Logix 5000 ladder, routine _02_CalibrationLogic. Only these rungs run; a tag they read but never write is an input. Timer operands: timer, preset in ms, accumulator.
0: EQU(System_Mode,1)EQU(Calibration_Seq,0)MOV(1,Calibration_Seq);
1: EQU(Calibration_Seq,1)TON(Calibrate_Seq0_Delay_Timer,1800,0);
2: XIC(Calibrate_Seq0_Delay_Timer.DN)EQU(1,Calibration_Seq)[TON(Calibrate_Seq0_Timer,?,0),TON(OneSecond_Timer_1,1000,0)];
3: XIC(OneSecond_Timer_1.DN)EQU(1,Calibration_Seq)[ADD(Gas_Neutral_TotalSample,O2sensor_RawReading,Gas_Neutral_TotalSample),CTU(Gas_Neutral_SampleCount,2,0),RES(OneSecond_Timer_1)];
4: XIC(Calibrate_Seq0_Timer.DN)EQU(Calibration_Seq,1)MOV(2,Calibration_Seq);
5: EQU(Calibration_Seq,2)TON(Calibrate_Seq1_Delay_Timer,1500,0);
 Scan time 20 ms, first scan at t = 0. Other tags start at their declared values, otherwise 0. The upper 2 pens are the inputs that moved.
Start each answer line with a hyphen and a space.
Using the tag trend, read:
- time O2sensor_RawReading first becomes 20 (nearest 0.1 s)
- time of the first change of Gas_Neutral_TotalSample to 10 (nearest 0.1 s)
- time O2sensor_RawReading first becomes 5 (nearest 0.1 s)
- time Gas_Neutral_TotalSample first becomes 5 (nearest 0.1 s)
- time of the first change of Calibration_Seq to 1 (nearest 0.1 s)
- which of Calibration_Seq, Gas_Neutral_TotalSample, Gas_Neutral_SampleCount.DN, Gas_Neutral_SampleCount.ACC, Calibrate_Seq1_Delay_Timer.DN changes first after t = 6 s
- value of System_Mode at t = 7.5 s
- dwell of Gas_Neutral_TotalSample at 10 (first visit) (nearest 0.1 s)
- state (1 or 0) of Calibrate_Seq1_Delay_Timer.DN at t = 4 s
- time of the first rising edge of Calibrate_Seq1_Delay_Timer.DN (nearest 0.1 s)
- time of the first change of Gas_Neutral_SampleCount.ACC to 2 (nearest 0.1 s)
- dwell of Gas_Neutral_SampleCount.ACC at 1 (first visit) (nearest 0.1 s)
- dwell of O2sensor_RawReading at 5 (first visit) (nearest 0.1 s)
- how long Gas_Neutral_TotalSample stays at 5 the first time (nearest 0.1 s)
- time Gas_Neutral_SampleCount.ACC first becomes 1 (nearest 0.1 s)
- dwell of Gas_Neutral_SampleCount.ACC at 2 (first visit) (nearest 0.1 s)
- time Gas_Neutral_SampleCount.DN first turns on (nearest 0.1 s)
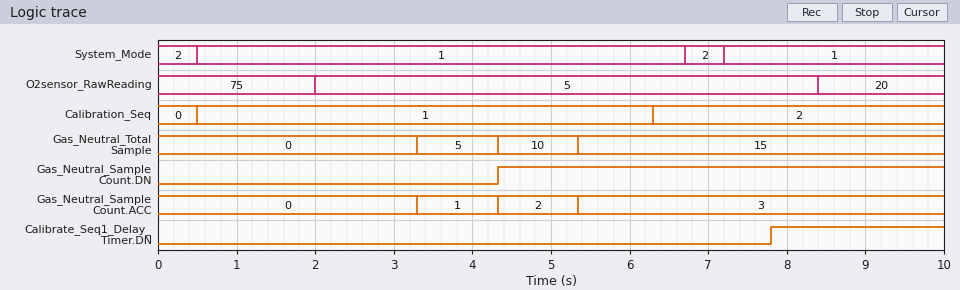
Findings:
- 8.4 s
- 4.3 s
- 2.0 s
- 3.3 s
- 0.5 s
- Calibration_Seq
- 1
- 1.0 s
- 0
- 7.8 s
- 4.3 s
- 1.0 s
- 6.4 s
- 1.0 s
- 3.3 s
- 1.0 s
- 4.3 s
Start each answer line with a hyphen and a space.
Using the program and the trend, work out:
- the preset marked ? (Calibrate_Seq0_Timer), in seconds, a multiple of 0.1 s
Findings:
- 4.0 s
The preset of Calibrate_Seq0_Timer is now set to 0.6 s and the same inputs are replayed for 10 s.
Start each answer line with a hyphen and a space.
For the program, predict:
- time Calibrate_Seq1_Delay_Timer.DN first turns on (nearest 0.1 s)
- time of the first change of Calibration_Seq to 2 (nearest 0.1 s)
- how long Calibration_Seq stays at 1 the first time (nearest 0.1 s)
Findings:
- 4.4 s
- 2.9 s
- 2.4 s
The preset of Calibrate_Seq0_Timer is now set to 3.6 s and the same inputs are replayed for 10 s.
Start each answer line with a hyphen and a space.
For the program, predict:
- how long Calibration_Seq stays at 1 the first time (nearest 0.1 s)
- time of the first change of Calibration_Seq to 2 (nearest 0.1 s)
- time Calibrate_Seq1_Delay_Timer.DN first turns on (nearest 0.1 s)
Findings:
- 5.4 s
- 5.9 s
- 7.4 s
